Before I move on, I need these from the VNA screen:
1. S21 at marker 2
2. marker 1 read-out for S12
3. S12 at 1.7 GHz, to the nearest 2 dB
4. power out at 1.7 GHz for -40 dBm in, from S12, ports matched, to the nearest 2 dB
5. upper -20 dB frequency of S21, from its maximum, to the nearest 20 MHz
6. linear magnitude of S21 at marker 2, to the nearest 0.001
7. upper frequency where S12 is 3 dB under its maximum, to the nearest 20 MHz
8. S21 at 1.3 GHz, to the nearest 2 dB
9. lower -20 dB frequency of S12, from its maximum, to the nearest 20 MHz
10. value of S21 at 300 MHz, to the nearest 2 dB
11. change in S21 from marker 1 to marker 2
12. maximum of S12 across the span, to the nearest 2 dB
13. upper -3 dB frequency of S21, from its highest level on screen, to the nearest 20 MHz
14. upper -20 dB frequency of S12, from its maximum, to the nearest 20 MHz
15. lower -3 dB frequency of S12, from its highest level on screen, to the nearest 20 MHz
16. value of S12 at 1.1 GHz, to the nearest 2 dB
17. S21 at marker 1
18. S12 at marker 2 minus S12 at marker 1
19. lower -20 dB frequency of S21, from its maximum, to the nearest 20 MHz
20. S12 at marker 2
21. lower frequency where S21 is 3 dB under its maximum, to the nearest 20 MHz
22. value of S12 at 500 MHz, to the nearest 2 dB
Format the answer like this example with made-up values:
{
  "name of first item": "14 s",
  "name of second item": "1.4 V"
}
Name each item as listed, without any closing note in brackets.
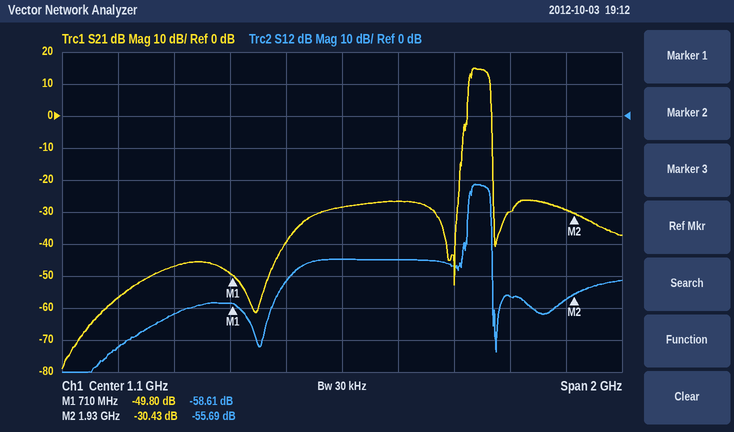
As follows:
{
  "S21 at marker 2": "-30.43 dB",
  "marker 1 read-out for S12": "-58.61 dB",
  "S12 at 1.7 GHz, to the nearest 2 dB": "-56 dB",
  "power out at 1.7 GHz for -40 dBm in, from S12, ports matched, to the nearest 2 dB": "-96 dBm",
  "upper -20 dB frequency of S21, from its maximum, to the nearest 20 MHz": "1.64 GHz",
  "linear magnitude of S21 at marker 2, to the nearest 0.001": "0.030",
  "upper frequency where S12 is 3 dB under its maximum, to the nearest 20 MHz": "1.62 GHz",
  "S21 at 1.3 GHz, to the nearest 2 dB": "-26 dB",
  "lower -20 dB frequency of S12, from its maximum, to the nearest 20 MHz": "1.54 GHz",
  "value of S21 at 300 MHz, to the nearest 2 dB": "-56 dB",
  "change in S21 from marker 1 to marker 2": "19.37 dB",
  "maximum of S12 across the span, to the nearest 2 dB": "-22 dB",
  "upper -3 dB frequency of S21, from its highest level on screen, to the nearest 20 MHz": "1.62 GHz",
  "upper -20 dB frequency of S12, from its maximum, to the nearest 20 MHz": "1.64 GHz",
  "lower -3 dB frequency of S12, from its highest level on screen, to the nearest 20 MHz": "1.56 GHz",
  "value of S12 at 1.1 GHz, to the nearest 2 dB": "-44 dB",
  "S21 at marker 1": "-49.80 dB",
  "S12 at marker 2 minus S12 at marker 1": "2.92 dB",
  "lower -20 dB frequency of S21, from its maximum, to the nearest 20 MHz": "1.54 GHz",
  "S12 at marker 2": "-55.69 dB",
  "lower frequency where S21 is 3 dB under its maximum, to the nearest 20 MHz": "1.56 GHz",
  "value of S12 at 500 MHz, to the nearest 2 dB": "-62 dB"
}
